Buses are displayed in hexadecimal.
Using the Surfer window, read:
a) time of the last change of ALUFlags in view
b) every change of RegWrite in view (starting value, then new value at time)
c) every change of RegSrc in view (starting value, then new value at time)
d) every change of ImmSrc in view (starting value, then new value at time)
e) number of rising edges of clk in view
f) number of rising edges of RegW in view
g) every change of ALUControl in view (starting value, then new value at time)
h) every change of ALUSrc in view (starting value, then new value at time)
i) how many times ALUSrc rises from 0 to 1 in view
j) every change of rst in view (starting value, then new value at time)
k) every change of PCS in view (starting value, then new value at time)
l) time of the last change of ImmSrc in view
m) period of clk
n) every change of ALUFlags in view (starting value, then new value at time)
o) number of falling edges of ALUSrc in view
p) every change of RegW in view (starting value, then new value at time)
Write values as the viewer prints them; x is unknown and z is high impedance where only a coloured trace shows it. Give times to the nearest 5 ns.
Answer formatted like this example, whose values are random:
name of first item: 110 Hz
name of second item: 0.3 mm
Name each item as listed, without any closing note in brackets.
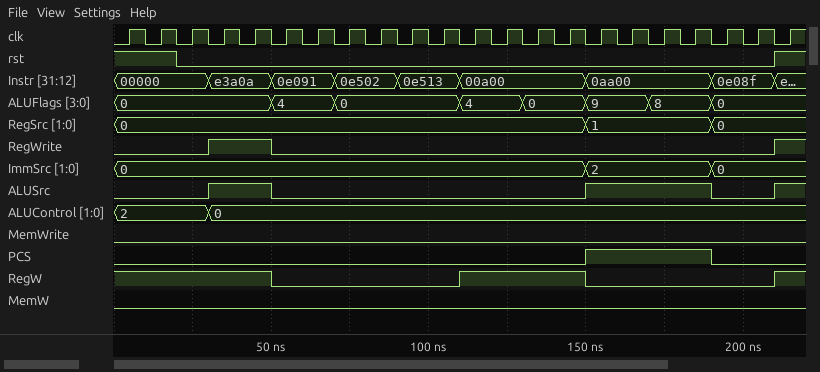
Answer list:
time of the last change of ALUFlags in view: 190 ns
every change of RegWrite in view: 0, 1 at 30 ns, 0 at 50 ns, 1 at 210 ns
every change of RegSrc in view: 0, 1 at 150 ns, 0 at 190 ns
every change of ImmSrc in view: 0, 2 at 150 ns, 0 at 190 ns
number of rising edges of clk in view: 22
number of rising edges of RegW in view: 2
every change of ALUControl in view: 2, 0 at 30 ns
every change of ALUSrc in view: 0, 1 at 30 ns, 0 at 50 ns, 1 at 150 ns, 0 at 190 ns, 1 at 210 ns
how many times ALUSrc rises from 0 to 1 in view: 3
every change of rst in view: 1, 0 at 20 ns, 1 at 210 ns
every change of PCS in view: 0, 1 at 150 ns, 0 at 190 ns
time of the last change of ImmSrc in view: 190 ns
period of clk: 10 ns
every change of ALUFlags in view: 0, 4 at 50 ns, 0 at 70 ns, 4 at 110 ns, 0 at 130 ns, 9 at 150 ns, 8 at 170 ns, 0 at 190 ns
number of falling edges of ALUSrc in view: 2
every change of RegW in view: 1, 0 at 50 ns, 1 at 110 ns, 0 at 150 ns, 1 at 210 ns
